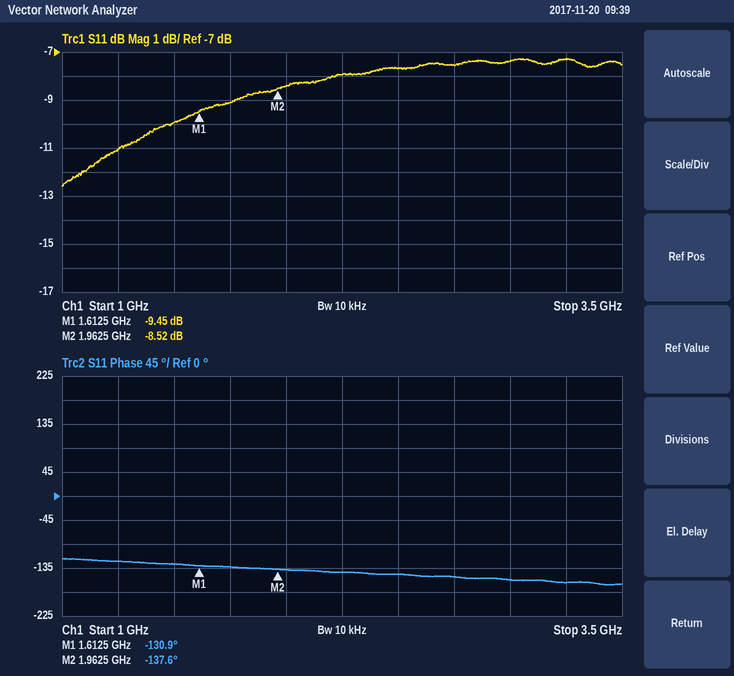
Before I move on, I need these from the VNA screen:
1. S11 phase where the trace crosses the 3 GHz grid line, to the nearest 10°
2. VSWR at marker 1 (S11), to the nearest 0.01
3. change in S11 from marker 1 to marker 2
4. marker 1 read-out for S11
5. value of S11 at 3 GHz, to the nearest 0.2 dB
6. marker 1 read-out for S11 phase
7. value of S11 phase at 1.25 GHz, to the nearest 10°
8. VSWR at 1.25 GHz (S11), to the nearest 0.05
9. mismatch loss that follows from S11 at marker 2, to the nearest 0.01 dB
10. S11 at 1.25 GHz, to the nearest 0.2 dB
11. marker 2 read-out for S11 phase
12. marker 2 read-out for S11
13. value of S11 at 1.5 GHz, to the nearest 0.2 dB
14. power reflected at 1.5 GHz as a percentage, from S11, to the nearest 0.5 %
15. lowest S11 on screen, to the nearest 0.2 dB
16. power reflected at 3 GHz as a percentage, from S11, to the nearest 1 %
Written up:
-160°
2.02
0.93 dB
-9.45 dB
-7.4 dB
-130.9°
-120°
1.80
0.66 dB
-11.0 dB
-137.6°
-8.52 dB
-10.0 dB
10.0 %
-12.6 dB
18 %
